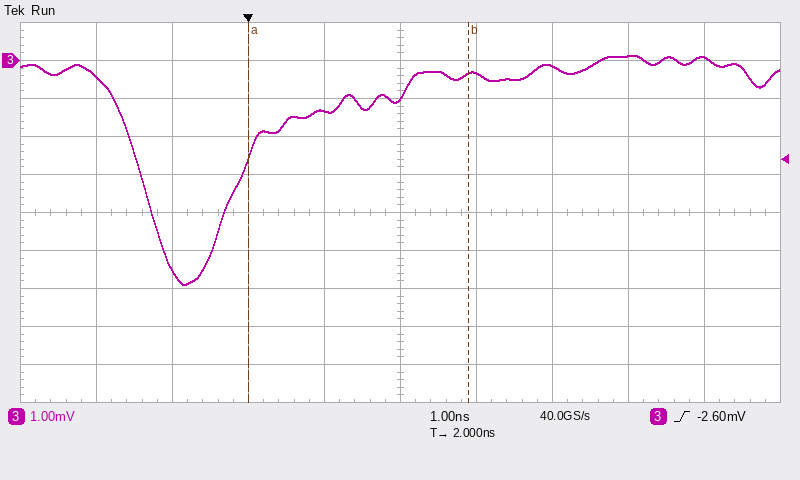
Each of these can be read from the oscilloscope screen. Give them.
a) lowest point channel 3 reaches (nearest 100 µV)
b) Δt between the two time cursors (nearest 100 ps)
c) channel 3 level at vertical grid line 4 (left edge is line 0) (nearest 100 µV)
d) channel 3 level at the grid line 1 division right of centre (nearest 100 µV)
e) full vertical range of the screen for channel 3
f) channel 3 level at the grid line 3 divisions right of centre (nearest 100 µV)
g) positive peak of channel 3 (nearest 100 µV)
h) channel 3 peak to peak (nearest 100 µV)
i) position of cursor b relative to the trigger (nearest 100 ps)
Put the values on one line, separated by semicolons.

-5.9 mV; 2.9 ns; -1.3 mV; -300 µV; 10 mV; 100 µV; 100 µV; 6.0 mV; +2.9 ns
